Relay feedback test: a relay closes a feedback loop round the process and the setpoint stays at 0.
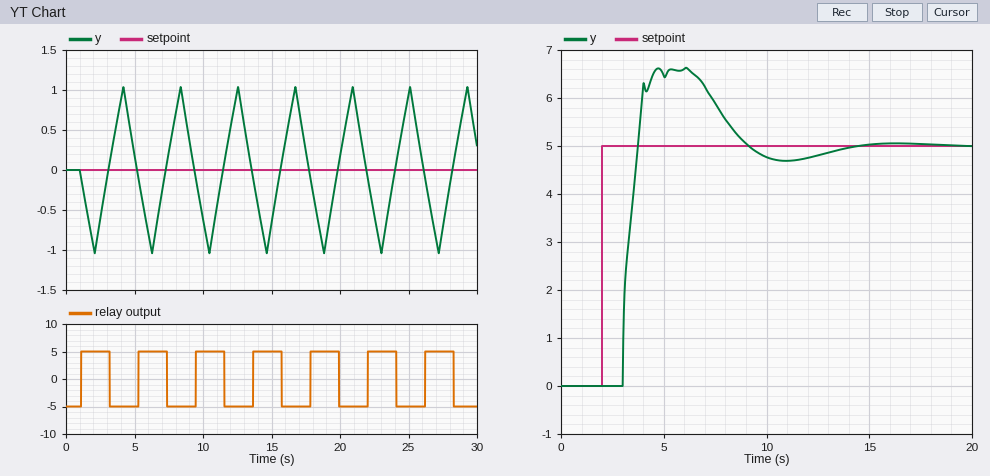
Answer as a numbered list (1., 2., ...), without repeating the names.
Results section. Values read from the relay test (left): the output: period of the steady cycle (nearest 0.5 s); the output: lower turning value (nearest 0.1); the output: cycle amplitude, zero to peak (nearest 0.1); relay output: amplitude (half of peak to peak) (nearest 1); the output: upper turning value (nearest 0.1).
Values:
1. 4.0 s
2. -1.0
3. 1.0
4. 5
5. 1.0
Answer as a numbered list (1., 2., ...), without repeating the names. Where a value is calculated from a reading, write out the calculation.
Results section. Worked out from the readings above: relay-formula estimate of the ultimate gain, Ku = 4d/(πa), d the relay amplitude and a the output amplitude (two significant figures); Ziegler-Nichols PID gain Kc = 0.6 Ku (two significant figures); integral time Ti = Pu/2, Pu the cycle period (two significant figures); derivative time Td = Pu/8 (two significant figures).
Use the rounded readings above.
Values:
1. 4 × 5 / (π × 1) = 6.4
2. 0.6 × 6.4 = 3.8
3. 4 / 2 = 2.0 s
4. 4 / 8 = 0.50 s
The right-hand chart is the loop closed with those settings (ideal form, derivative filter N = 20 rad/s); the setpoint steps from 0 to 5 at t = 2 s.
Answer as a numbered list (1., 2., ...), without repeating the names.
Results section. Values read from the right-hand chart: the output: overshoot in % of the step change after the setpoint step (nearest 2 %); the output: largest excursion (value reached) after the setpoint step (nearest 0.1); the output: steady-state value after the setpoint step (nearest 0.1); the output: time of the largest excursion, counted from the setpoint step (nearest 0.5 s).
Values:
1. 32 %
2. 6.6
3. 5.0
4. 4.0 s
